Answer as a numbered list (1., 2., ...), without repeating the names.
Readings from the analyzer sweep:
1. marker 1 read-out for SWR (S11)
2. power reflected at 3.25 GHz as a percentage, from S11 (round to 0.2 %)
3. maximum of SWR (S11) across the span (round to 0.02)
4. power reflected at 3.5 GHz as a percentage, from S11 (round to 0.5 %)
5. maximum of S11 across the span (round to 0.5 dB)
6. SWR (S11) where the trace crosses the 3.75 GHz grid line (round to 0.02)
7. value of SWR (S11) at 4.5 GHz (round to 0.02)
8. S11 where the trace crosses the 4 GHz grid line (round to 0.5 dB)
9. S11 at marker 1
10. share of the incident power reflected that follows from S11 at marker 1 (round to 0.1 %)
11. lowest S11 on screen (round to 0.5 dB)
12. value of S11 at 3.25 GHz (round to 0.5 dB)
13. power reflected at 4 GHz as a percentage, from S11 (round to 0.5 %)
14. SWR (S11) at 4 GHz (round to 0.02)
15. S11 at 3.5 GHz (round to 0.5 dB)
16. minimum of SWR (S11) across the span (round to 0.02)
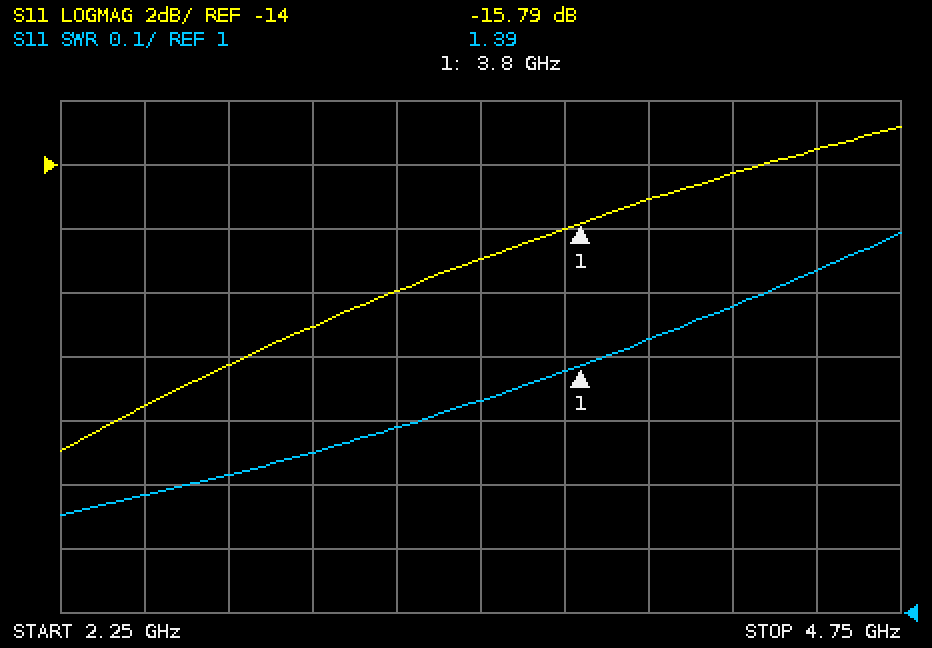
1. 1.39
2. 1.6 %
3. 1.60
4. 2.0 %
5. -13.0 dB
6. 1.38
7. 1.54
8. -15.0 dB
9. -15.79 dB
10. 2.6 %
11. -23.0 dB
12. -18.0 dB
13. 3.0 %
14. 1.42
15. -17.0 dB
16. 1.16
